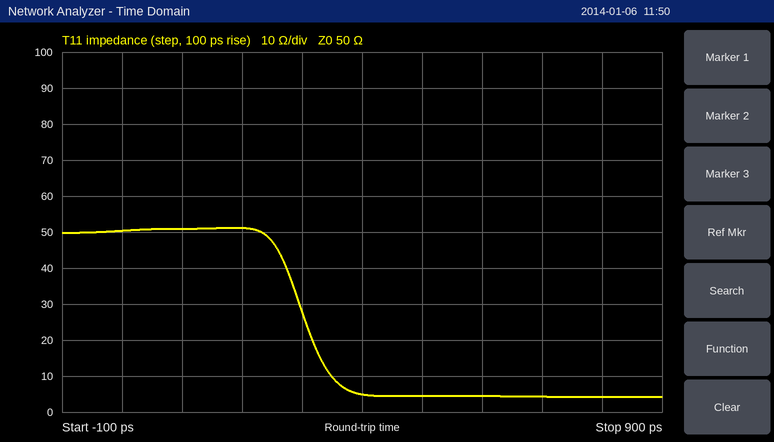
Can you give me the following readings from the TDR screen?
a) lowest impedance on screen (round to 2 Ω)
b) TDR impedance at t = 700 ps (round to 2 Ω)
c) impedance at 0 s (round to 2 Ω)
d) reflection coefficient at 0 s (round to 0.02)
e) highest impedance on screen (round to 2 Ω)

4 Ω
4 Ω
50 Ω
0.00
52 Ω
